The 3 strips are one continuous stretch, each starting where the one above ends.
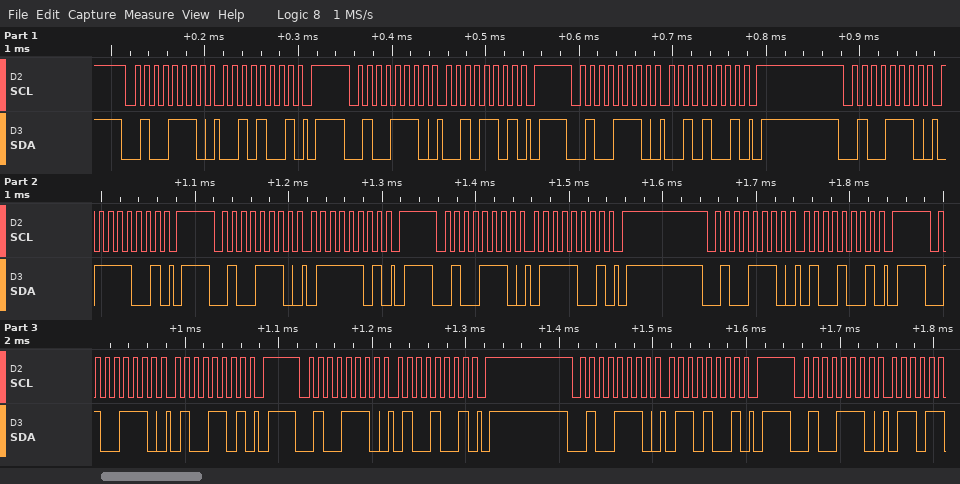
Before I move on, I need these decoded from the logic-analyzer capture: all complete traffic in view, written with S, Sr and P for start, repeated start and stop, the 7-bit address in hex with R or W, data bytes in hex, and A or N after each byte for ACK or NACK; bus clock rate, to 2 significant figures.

S 27W A 29 A P S 27W A 2D A P S 27W A 29 A P S 27W A 79 A P S 27W A 7D A P S 27W A 79 A P S 27W A 49 A P S 27W A 4D A P S 27W A 49 A P S 27W A 69 A P S 27W A
100 kHz
